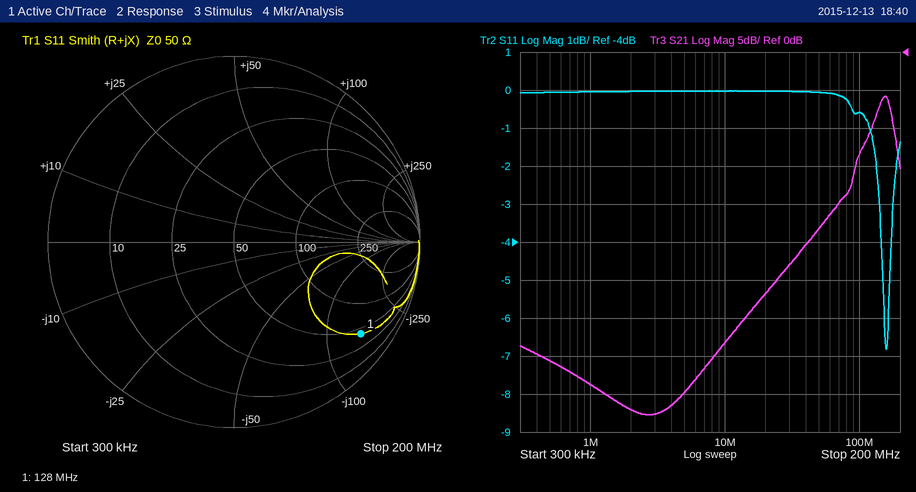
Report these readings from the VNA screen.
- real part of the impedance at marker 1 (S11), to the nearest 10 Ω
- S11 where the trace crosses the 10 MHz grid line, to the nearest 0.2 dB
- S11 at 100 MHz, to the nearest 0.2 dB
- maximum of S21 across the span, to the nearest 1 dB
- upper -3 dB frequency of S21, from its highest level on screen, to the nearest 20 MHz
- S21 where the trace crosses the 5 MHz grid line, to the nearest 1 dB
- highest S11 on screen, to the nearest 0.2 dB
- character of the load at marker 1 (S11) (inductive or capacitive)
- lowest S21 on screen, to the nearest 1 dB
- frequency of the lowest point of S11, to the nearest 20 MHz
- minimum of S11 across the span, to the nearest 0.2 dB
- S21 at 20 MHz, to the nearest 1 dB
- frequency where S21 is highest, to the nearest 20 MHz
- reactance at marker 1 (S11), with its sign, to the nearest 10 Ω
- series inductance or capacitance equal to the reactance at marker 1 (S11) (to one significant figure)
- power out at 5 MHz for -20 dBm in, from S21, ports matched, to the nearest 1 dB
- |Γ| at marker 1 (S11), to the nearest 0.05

40 Ω
0.0 dB
-0.6 dB
-6 dB
180 MHz
-45 dB
0.0 dB
capacitive
-48 dB
160 MHz
-6.8 dB
-32 dB
160 MHz
-140 Ω
9 pF
-65 dBm
0.85
